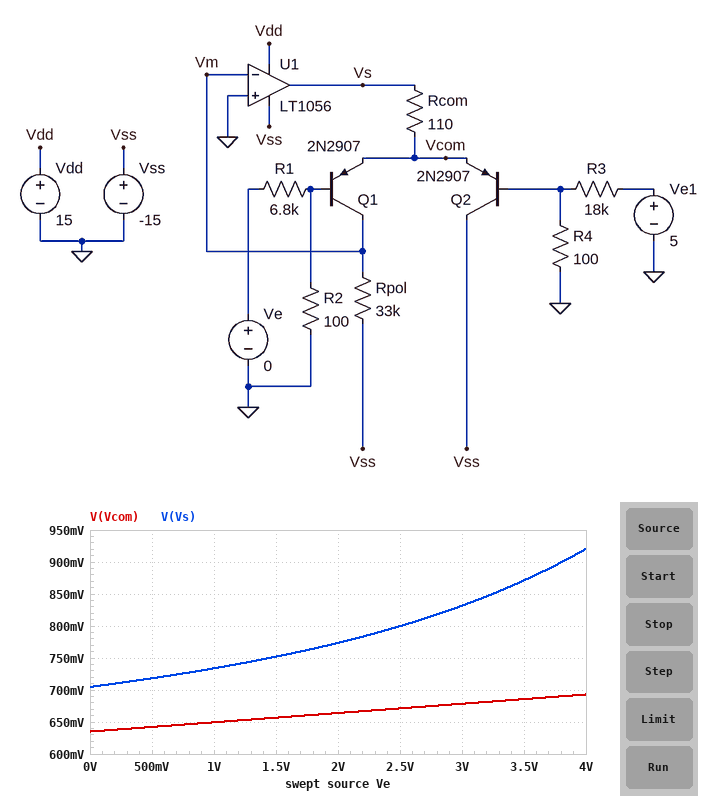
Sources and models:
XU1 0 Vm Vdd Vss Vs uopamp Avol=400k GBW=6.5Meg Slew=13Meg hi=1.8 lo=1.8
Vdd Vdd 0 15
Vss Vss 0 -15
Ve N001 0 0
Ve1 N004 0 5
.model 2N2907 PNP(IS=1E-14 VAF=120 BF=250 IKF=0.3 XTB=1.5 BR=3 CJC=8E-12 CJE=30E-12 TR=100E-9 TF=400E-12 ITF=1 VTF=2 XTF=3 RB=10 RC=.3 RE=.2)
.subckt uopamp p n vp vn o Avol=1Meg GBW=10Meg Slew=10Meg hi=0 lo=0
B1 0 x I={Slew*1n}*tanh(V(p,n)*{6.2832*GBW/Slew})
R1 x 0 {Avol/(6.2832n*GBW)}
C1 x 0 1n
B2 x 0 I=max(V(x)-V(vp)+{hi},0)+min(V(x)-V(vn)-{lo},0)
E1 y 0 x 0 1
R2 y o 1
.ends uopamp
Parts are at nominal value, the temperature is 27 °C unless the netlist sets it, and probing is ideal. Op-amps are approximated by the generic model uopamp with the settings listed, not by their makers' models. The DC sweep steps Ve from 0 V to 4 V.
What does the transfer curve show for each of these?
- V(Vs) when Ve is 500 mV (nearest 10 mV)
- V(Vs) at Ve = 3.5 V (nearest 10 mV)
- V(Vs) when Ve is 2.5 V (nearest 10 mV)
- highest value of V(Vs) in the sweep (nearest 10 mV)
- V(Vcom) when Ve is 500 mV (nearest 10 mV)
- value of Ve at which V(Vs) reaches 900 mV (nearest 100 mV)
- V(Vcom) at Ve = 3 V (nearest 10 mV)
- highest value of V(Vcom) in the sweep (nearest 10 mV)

720 mV
870 mV
800 mV
920 mV
640 mV
3.8 V
680 mV
690 mV
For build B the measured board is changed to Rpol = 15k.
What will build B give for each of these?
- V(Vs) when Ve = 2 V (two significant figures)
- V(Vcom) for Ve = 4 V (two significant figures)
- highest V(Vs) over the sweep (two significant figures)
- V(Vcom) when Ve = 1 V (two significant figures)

930 mV
710 mV
1.2 V
670 mV
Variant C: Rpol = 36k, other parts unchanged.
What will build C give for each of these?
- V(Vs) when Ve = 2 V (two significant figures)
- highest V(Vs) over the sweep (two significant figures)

760 mV
900 mV
